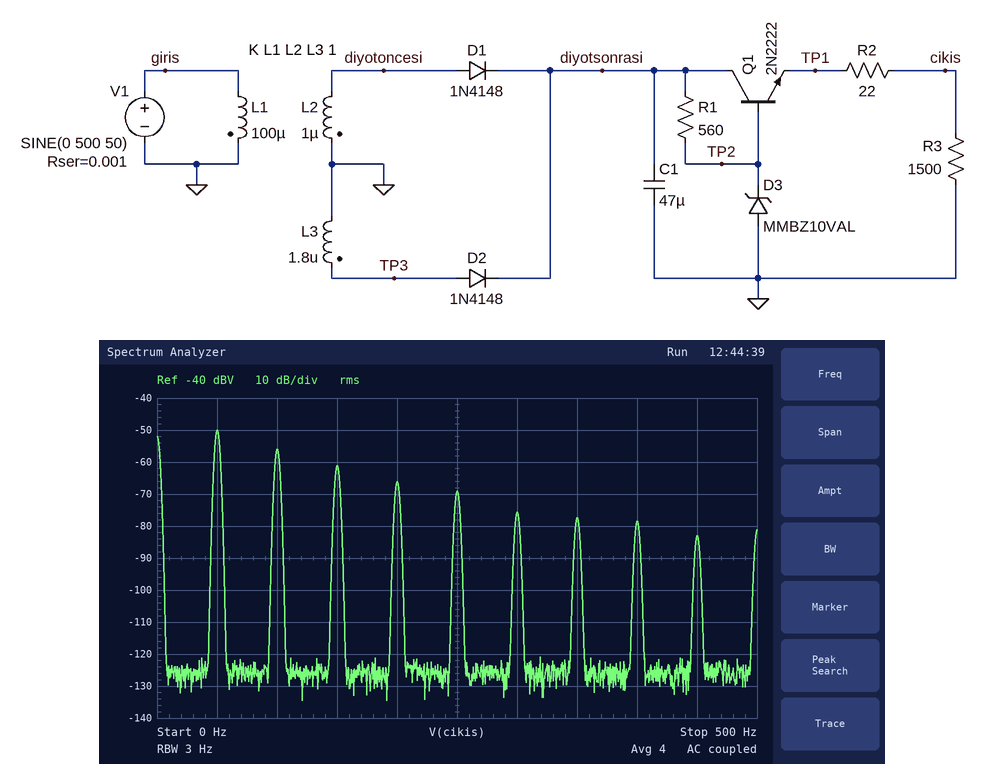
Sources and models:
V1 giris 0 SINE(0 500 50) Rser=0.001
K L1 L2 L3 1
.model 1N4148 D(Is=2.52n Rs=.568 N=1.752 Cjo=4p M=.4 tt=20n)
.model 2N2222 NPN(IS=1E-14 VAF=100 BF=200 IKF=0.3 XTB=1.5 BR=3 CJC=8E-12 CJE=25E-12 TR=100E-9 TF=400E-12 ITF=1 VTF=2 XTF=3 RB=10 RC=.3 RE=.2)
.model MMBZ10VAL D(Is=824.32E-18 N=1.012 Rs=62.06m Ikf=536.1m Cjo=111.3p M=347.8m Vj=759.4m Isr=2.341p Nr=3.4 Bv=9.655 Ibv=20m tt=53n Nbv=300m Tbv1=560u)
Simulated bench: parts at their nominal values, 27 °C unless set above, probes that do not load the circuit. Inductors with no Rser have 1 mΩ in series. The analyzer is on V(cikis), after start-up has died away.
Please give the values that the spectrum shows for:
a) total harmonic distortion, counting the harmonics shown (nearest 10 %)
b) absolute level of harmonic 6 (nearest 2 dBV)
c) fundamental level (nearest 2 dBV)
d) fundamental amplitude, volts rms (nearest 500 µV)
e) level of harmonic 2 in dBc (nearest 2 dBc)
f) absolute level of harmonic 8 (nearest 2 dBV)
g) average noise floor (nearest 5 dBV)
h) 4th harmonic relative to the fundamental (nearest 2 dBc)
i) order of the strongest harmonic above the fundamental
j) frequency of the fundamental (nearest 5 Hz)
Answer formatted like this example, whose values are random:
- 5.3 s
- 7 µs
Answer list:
- 60 %
- -76 dBV
- -50 dBV
- 3.0 mV
- -6 dBc
- -78 dBV
- -125 dBV
- -16 dBc
- 2
- 50 Hz
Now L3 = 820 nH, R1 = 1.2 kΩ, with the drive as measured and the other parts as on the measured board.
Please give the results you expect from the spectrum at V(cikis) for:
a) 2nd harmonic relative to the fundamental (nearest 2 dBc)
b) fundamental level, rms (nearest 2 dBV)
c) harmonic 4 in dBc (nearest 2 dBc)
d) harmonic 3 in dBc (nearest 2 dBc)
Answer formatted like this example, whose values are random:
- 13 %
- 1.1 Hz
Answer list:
- -2 dBc
- -60 dBV
- -10 dBc
- -10 dBc
